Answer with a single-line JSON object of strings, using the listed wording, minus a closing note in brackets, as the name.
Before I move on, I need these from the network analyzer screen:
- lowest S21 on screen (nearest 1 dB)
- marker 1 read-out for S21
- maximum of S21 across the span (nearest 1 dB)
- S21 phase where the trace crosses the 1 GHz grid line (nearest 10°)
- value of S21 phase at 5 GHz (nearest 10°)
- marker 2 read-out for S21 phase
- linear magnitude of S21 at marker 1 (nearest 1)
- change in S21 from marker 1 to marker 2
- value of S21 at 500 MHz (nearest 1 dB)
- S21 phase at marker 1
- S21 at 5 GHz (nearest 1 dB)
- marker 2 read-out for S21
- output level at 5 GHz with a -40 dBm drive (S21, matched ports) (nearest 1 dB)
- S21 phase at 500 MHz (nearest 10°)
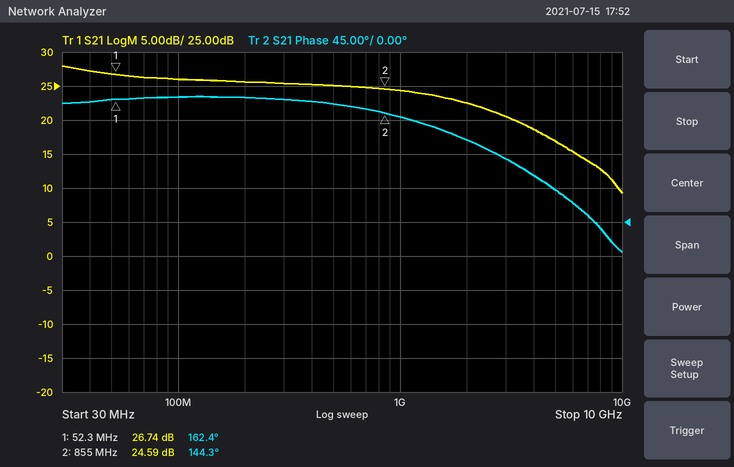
{"lowest S21 on screen": "9 dB", "marker 1 read-out for S21": "26.74 dB", "maximum of S21 across the span": "28 dB", "S21 phase where the trace crosses the 1 GHz grid line": "140°", "value of S21 phase at 5 GHz": "40°", "marker 2 read-out for S21 phase": "144.3°", "linear magnitude of S21 at marker 1": "22", "change in S21 from marker 1 to marker 2": "-2.15 dB", "value of S21 at 500 MHz": "25 dB", "S21 phase at marker 1": "162.4°", "S21 at 5 GHz": "17 dB", "marker 2 read-out for S21": "24.59 dB", "output level at 5 GHz with a -40 dBm drive (S21, matched ports)": "-23 dBm", "S21 phase at 500 MHz": "160°"}
